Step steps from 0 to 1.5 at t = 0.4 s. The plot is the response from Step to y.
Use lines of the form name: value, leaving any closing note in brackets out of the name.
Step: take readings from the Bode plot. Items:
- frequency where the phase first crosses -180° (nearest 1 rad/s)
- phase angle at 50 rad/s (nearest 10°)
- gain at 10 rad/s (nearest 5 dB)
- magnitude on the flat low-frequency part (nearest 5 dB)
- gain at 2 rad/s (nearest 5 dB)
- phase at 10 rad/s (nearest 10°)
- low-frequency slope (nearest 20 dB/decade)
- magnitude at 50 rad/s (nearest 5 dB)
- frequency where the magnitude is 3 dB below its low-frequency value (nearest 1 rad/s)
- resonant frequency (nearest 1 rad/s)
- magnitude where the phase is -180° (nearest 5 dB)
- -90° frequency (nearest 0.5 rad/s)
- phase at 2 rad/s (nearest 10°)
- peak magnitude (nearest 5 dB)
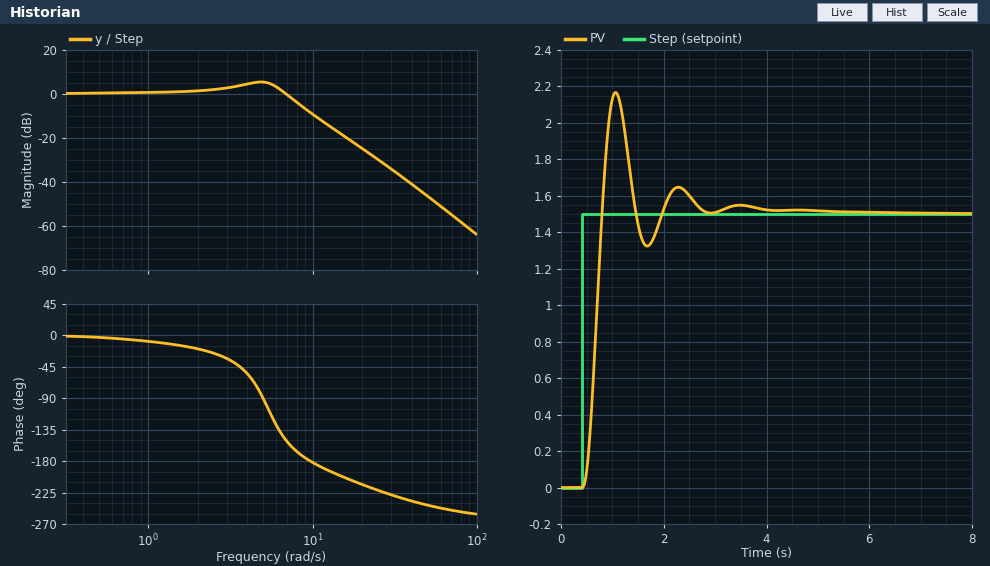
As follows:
frequency where the phase first crosses -180°: 10 rad/s
phase angle at 50 rad/s: -240°
gain at 10 rad/s: -10 dB
magnitude on the flat low-frequency part: 0 dB
gain at 2 rad/s: 0 dB
phase at 10 rad/s: -180°
low-frequency slope: 0 dB/decade
magnitude at 50 rad/s: -45 dB
frequency where the magnitude is 3 dB below its low-frequency value: 8 rad/s
resonant frequency: 5 rad/s
magnitude where the phase is -180°: -10 dB
-90° frequency: 5.0 rad/s
phase at 2 rad/s: -20°
peak magnitude: 5 dB
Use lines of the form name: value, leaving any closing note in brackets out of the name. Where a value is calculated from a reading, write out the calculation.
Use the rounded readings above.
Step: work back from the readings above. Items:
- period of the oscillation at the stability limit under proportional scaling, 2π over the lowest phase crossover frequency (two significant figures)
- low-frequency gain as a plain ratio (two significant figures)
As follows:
period of the oscillation at the stability limit under proportional scaling, 2π over the lowest phase crossover frequency: 2π / 10 = 0.63 s
low-frequency gain as a plain ratio: 10^(0 / 20) = 1.0
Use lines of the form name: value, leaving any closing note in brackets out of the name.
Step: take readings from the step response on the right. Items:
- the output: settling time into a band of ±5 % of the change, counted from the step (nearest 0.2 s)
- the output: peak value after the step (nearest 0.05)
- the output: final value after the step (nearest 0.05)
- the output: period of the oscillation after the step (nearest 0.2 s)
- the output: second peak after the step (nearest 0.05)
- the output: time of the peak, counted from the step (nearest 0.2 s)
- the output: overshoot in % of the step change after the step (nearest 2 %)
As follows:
the output: settling time into a band of ±5 % of the change, counted from the step: 2.2 s
the output: peak value after the step: 2.15
the output: final value after the step: 1.50
the output: period of the oscillation after the step: 1.2 s
the output: second peak after the step: 1.65
the output: time of the peak, counted from the step: 0.6 s
the output: overshoot in % of the step change after the step: 44 %
